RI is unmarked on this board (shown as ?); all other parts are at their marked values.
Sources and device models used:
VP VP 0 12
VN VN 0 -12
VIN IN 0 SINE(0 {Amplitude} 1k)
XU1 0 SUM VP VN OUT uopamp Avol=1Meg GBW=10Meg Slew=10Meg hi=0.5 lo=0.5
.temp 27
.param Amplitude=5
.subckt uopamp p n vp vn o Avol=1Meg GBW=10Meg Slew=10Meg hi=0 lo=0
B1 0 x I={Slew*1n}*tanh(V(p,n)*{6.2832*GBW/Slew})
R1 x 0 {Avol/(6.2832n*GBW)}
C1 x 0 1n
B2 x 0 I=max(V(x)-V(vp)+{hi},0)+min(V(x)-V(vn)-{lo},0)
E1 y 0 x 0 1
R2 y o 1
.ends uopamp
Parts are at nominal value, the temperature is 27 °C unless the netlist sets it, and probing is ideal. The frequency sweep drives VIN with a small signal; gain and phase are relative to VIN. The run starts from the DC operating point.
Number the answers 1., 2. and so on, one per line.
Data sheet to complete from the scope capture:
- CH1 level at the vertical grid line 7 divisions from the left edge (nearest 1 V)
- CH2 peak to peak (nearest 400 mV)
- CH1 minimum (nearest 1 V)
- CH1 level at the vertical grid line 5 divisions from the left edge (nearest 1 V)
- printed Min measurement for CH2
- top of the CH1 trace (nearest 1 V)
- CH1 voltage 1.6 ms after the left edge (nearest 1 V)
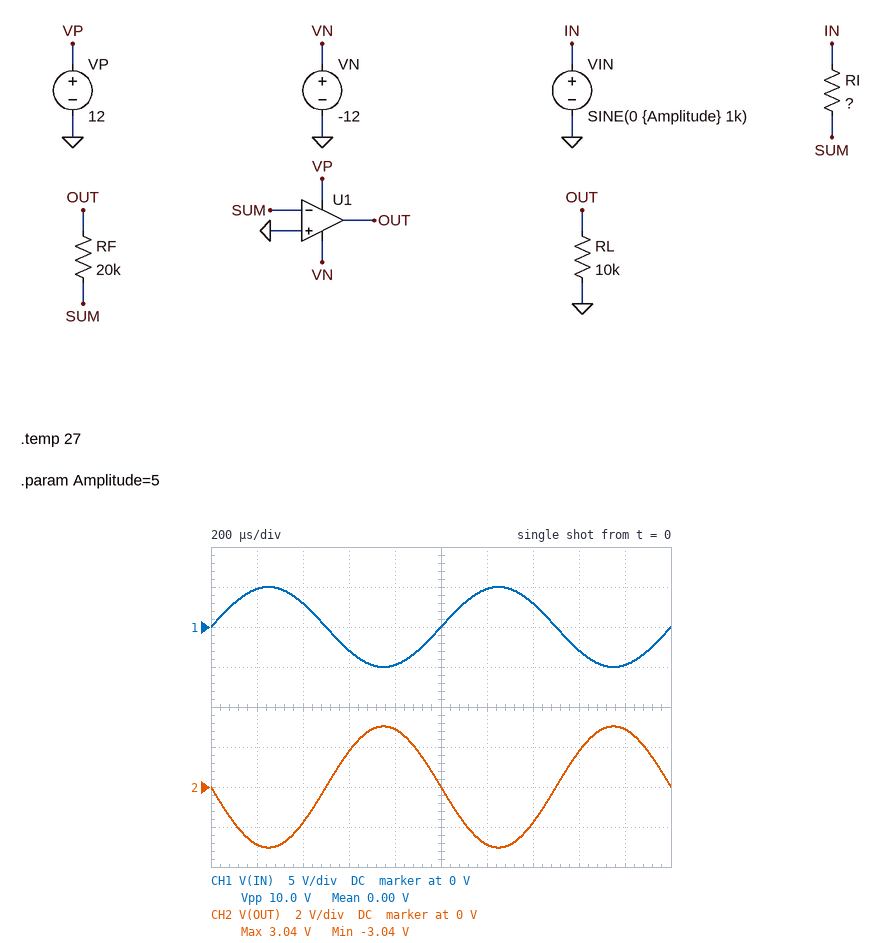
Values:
1. 3 V
2. 6.0 V
3. -5 V
4. 0 V
5. -3.04 V
6. 5 V
7. -3 V
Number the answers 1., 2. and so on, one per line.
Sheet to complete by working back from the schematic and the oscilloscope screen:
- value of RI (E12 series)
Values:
1. 33 kΩ
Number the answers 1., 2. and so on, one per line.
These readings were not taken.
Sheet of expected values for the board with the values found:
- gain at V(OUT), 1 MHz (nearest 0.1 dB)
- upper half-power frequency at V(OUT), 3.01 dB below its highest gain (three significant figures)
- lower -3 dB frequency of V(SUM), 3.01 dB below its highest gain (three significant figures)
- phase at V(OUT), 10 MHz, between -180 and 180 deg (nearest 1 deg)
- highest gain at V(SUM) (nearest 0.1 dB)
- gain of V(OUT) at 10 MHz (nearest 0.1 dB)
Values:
1. -4.5 dB
2. 6.23 MHz
3. 6.23 MHz
4. 122 deg
5. -8.5 dB
6. -9.9 dB
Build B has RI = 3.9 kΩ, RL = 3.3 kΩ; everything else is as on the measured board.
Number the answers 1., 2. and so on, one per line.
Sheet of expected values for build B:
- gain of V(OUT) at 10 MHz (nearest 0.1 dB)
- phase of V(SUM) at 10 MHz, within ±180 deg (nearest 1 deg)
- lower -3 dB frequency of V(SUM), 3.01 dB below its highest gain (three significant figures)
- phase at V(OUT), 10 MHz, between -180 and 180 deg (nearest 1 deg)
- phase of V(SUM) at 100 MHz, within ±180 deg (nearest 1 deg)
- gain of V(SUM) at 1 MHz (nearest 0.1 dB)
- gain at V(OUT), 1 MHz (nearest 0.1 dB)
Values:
1. -1.7 dB
2. 9 deg
3. 1.63 MHz
4. 99 deg
5. 1 deg
6. -7.2 dB
7. 12.8 dB
